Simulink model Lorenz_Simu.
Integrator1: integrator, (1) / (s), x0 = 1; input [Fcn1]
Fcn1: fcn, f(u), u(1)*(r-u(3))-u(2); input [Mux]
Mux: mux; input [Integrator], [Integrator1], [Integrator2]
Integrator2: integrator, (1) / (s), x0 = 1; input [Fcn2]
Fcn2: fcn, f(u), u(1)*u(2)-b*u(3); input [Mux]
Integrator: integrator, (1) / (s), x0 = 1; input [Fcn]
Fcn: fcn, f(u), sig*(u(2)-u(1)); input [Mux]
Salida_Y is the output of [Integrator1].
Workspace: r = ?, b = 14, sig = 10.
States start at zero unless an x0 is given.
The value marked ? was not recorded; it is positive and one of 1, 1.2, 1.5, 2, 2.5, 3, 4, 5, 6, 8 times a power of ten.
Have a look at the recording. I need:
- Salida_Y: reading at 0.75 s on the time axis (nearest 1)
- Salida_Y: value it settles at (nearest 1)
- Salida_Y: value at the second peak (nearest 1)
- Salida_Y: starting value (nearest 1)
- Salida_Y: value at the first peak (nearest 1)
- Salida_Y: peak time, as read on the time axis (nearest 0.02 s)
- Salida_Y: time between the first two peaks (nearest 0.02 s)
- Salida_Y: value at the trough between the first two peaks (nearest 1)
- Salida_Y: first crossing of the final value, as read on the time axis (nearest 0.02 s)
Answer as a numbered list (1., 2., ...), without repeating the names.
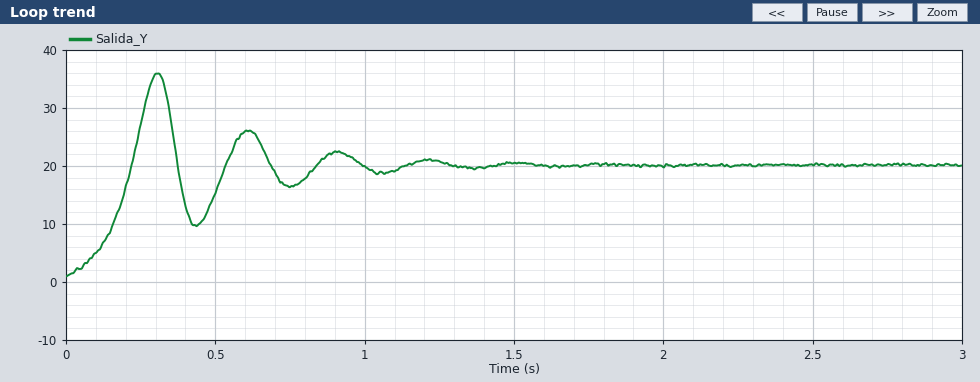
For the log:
1. 16
2. 20
3. 26
4. 1
5. 36
6. 0.30 s
7. 0.30 s
8. 10
9. 0.22 s
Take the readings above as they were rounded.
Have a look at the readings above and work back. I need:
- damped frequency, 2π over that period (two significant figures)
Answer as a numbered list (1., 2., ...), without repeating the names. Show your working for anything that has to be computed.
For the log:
1. 2π / 0.3 = 21 rad/s
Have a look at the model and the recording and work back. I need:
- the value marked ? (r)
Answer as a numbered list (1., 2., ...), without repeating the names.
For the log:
1. 30
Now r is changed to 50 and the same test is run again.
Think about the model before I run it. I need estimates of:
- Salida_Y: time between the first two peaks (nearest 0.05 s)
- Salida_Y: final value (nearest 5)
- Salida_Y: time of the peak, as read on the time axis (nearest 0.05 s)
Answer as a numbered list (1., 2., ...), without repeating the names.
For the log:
1. 0.25 s
2. 25
3. 0.25 s
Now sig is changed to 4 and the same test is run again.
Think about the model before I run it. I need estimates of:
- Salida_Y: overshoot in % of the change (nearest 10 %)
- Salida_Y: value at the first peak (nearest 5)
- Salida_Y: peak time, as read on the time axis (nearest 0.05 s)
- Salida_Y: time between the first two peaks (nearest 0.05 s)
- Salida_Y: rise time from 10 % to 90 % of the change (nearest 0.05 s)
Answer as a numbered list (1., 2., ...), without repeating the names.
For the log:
1. 90 %
2. 40
3. 0.40 s
4. 0.35 s
5. 0.20 s
